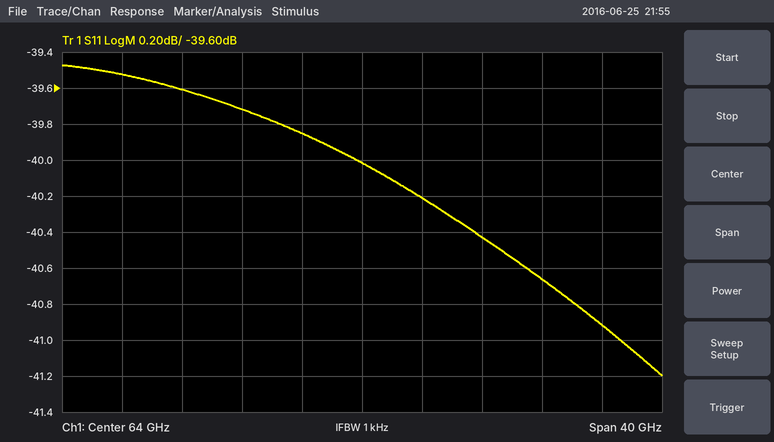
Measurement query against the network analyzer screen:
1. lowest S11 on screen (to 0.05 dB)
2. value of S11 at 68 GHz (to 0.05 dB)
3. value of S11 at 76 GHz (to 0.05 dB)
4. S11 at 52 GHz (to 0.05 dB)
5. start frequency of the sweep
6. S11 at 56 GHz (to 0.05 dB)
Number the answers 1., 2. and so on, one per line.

1. -41.20 dB
2. -40.20 dB
3. -40.65 dB
4. -39.60 dB
5. 44 GHz
6. -39.70 dB
